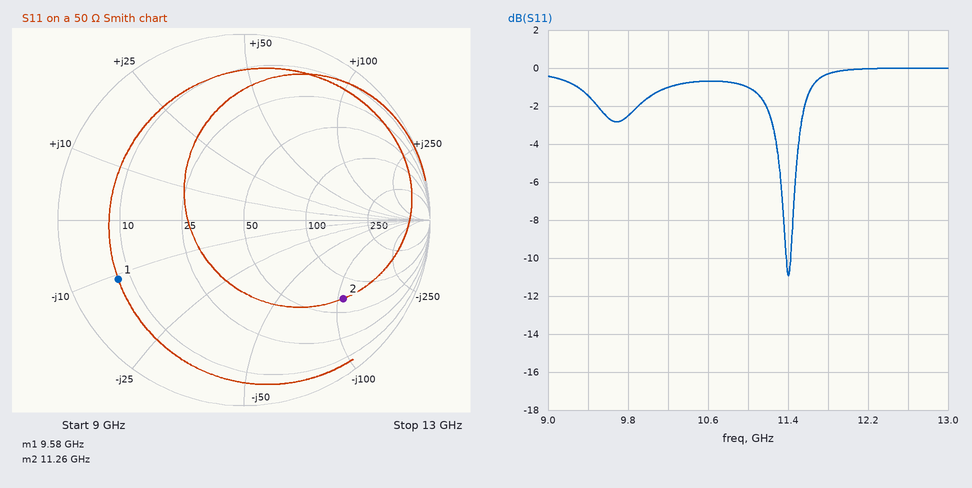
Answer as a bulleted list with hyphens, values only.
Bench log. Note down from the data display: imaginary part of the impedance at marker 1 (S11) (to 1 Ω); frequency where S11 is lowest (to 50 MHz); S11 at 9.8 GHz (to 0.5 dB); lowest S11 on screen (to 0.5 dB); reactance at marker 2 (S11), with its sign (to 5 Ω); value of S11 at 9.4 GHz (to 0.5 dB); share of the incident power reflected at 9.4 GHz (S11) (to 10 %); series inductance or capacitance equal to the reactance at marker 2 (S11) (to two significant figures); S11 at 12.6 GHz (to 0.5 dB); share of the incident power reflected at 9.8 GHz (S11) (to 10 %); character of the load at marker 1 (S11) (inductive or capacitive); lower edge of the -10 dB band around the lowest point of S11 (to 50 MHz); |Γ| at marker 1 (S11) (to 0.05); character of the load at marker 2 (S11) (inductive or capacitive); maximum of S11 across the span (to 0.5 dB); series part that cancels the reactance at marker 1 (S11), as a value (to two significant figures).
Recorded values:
- -11 Ω
- 11.40 GHz
- -2.5 dB
- -11.0 dB
- -105 Ω
- -1.5 dB
- 70 %
- 130 fF
- 0.0 dB
- 60 %
- capacitive
- 11.40 GHz
- 0.75
- capacitive
- 0.0 dB
- 180 pH
